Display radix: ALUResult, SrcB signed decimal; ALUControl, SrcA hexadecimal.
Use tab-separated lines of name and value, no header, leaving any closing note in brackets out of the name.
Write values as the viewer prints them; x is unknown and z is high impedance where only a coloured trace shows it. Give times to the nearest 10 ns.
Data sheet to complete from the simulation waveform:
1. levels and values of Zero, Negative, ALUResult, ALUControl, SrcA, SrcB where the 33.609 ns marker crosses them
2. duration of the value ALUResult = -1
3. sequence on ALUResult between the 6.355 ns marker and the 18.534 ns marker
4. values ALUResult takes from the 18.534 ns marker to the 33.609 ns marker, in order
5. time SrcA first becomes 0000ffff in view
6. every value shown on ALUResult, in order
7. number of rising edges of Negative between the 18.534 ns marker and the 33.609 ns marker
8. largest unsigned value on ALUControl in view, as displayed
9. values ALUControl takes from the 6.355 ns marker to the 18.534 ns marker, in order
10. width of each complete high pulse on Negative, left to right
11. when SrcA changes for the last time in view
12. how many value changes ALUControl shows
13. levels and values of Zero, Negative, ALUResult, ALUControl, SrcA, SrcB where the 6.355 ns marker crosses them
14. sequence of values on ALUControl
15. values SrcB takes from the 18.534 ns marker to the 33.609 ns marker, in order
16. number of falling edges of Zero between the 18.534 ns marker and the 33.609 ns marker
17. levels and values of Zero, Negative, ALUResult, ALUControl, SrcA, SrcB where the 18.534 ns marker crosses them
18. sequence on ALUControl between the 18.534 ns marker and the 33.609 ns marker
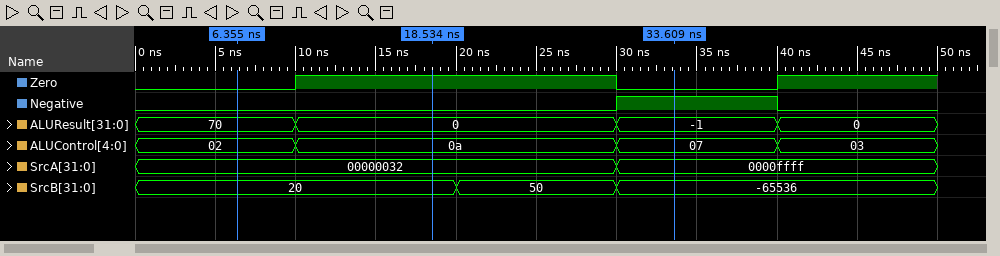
levels and values of Zero, Negative, ALUResult, ALUControl, SrcA, SrcB where the 33.609 ns marker crosses them	Zero=0, Negative=1, ALUResult=-1, ALUControl=07, SrcA=0000ffff, SrcB=-65536
duration of the value ALUResult = -1	10 ns
sequence on ALUResult between the 6.355 ns marker and the 18.534 ns marker	70, 0
values ALUResult takes from the 18.534 ns marker to the 33.609 ns marker, in order	0, -1
time SrcA first becomes 0000ffff in view	30 ns
every value shown on ALUResult, in order	70, 0, -1, 0
number of rising edges of Negative between the 18.534 ns marker and the 33.609 ns marker	1
largest unsigned value on ALUControl in view, as displayed	0a
values ALUControl takes from the 6.355 ns marker to the 18.534 ns marker, in order	02, 0a
width of each complete high pulse on Negative, left to right	10 ns
when SrcA changes for the last time in view	30 ns
how many value changes ALUControl shows	3
levels and values of Zero, Negative, ALUResult, ALUControl, SrcA, SrcB where the 6.355 ns marker crosses them	Zero=0, Negative=0, ALUResult=70, ALUControl=02, SrcA=00000032, SrcB=20
sequence of values on ALUControl	02, 0a, 07, 03
values SrcB takes from the 18.534 ns marker to the 33.609 ns marker, in order	20, 50, -65536
number of falling edges of Zero between the 18.534 ns marker and the 33.609 ns marker	1
levels and values of Zero, Negative, ALUResult, ALUControl, SrcA, SrcB where the 18.534 ns marker crosses them	Zero=1, Negative=0, ALUResult=0, ALUControl=0a, SrcA=00000032, SrcB=20
sequence on ALUControl between the 18.534 ns marker and the 33.609 ns marker	0a, 07
